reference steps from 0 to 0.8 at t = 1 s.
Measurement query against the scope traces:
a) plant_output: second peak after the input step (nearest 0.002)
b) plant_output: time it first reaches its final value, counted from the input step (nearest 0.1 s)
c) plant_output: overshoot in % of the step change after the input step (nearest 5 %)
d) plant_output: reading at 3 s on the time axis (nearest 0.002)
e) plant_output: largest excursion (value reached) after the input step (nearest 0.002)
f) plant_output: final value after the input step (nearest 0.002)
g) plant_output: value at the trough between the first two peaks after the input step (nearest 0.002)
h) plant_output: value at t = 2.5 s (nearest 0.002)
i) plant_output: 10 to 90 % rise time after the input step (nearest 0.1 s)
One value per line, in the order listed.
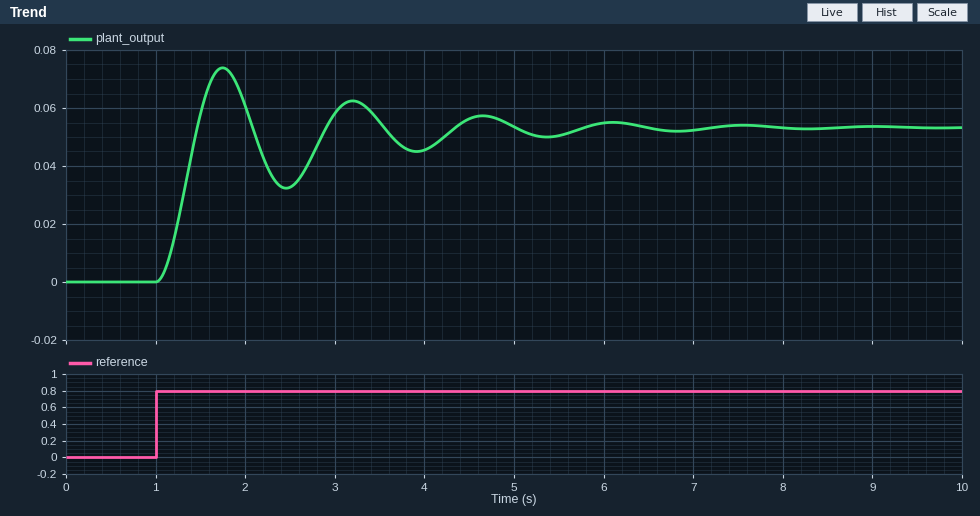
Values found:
0.062
0.5 s
40 %
0.058
0.074
0.054
0.032
0.032
0.3 s
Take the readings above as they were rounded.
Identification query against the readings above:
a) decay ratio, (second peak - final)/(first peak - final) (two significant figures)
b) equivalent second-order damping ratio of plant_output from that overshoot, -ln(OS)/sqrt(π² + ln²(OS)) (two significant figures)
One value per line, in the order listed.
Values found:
0.40
0.28
